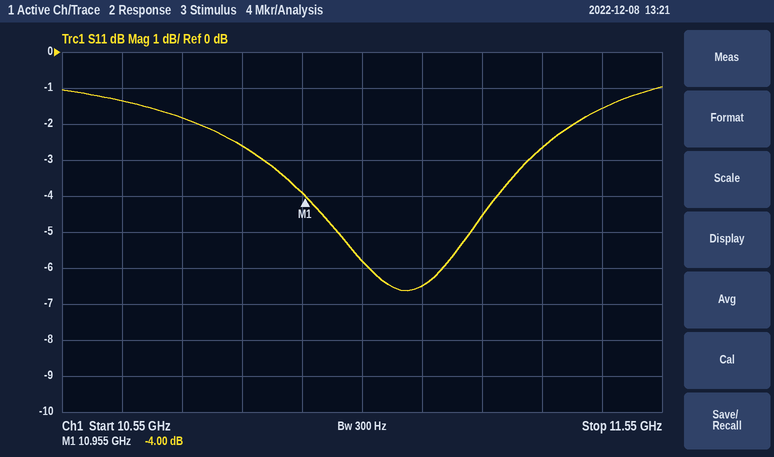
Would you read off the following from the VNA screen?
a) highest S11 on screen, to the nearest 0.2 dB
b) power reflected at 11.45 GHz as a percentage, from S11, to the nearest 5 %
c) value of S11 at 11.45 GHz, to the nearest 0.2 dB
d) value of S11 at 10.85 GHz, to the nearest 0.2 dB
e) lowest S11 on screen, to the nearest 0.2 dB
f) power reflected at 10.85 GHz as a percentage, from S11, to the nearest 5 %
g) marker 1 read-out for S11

-1.0 dB
70 %
-1.6 dB
-2.6 dB
-6.6 dB
55 %
-4.00 dB
